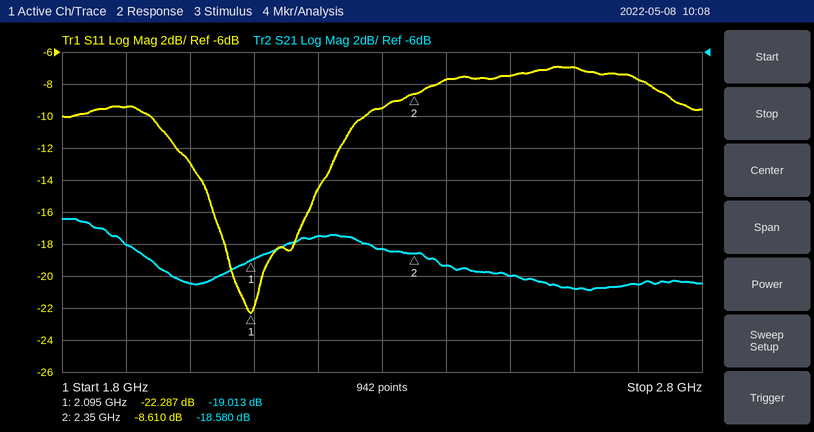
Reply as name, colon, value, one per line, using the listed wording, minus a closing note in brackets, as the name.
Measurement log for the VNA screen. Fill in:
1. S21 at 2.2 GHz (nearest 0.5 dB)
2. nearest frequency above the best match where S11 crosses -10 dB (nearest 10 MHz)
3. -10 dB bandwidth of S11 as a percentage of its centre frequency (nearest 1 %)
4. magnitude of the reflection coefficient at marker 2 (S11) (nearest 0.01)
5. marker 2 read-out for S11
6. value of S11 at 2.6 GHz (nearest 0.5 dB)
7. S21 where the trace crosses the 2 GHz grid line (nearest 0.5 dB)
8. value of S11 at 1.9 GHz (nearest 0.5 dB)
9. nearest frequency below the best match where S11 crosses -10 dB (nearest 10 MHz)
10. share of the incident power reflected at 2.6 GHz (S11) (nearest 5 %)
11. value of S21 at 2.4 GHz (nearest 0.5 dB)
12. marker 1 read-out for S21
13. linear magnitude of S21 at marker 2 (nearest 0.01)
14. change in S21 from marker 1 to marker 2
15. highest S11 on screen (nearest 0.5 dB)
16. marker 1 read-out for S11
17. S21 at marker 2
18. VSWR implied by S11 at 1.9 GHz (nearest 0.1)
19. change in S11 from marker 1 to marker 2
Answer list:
S21 at 2.2 GHz: -17.5 dB
nearest frequency above the best match where S11 crosses -10 dB: 2.27 GHz
-10 dB bandwidth of S11 as a percentage of its centre frequency: 16 %
magnitude of the reflection coefficient at marker 2 (S11): 0.37
marker 2 read-out for S11: -8.610 dB
value of S11 at 2.6 GHz: -7.0 dB
S21 where the trace crosses the 2 GHz grid line: -20.5 dB
value of S11 at 1.9 GHz: -9.5 dB
nearest frequency below the best match where S11 crosses -10 dB: 1.94 GHz
share of the incident power reflected at 2.6 GHz (S11): 20 %
value of S21 at 2.4 GHz: -19.5 dB
marker 1 read-out for S21: -19.013 dB
linear magnitude of S21 at marker 2: 0.12
change in S21 from marker 1 to marker 2: 0.433 dB
highest S11 on screen: -7.0 dB
marker 1 read-out for S11: -22.287 dB
S21 at marker 2: -18.580 dB
VSWR implied by S11 at 1.9 GHz: 2.0
change in S11 from marker 1 to marker 2: 13.677 dB
